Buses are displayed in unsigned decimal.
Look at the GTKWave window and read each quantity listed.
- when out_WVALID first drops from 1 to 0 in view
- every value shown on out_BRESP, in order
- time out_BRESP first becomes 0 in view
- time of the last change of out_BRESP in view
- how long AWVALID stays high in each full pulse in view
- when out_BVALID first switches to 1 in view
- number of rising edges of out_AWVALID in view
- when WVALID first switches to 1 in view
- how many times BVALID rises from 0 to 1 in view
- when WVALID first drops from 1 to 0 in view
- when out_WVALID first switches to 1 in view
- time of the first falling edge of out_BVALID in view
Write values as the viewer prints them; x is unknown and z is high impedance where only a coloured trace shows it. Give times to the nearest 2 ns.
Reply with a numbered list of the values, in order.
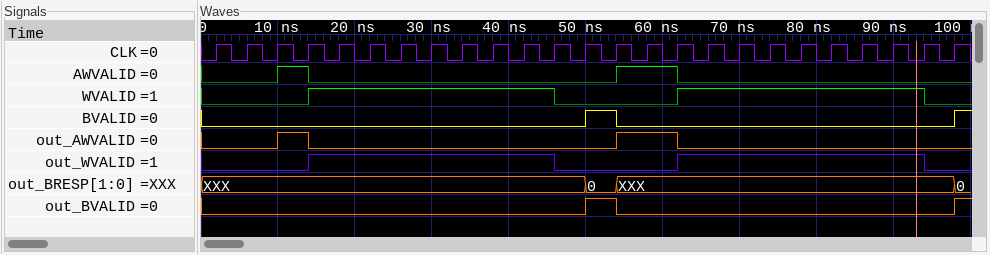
1. 46 ns
2. XXX, 0, XXX, 0
3. 50 ns
4. 98 ns
5. 4 ns, 8 ns
6. 50 ns
7. 2
8. 14 ns
9. 2
10. 46 ns
11. 14 ns
12. 54 ns
